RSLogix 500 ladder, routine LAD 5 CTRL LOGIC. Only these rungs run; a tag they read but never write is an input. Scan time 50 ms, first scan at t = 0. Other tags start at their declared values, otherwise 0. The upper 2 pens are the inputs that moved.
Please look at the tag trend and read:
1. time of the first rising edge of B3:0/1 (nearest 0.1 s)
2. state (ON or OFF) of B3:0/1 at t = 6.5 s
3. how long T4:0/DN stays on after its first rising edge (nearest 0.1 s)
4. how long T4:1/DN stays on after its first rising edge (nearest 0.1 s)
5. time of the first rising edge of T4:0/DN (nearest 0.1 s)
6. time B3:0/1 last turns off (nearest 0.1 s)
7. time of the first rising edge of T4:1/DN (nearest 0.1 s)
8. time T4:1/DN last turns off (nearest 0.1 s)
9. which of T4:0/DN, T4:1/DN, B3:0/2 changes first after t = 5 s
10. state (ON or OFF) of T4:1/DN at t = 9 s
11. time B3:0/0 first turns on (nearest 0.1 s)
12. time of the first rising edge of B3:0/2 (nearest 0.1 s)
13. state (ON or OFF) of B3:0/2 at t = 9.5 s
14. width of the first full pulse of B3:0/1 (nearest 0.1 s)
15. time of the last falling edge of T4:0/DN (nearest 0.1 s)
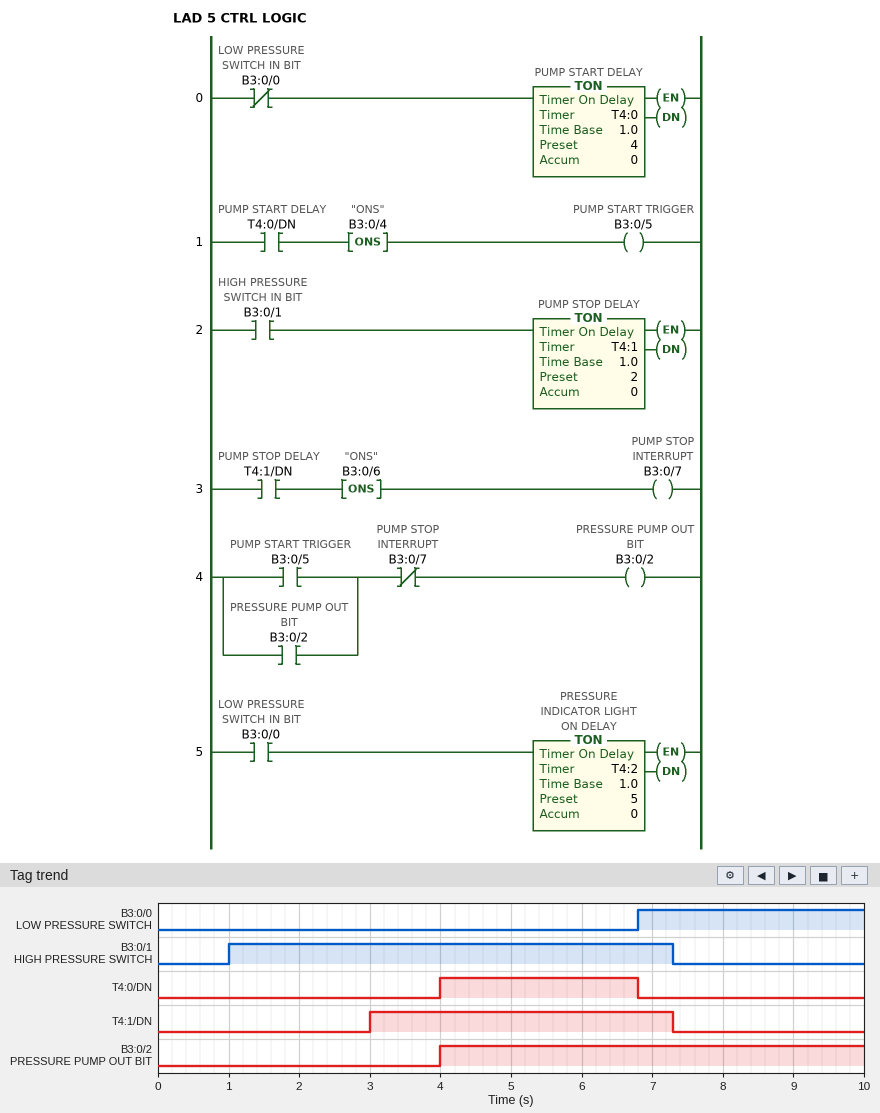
1.0 s
ON
2.8 s
4.3 s
4.0 s
7.3 s
3.0 s
7.3 s
T4:0/DN
OFF
6.8 s
4.0 s
ON
6.3 s
6.8 s
